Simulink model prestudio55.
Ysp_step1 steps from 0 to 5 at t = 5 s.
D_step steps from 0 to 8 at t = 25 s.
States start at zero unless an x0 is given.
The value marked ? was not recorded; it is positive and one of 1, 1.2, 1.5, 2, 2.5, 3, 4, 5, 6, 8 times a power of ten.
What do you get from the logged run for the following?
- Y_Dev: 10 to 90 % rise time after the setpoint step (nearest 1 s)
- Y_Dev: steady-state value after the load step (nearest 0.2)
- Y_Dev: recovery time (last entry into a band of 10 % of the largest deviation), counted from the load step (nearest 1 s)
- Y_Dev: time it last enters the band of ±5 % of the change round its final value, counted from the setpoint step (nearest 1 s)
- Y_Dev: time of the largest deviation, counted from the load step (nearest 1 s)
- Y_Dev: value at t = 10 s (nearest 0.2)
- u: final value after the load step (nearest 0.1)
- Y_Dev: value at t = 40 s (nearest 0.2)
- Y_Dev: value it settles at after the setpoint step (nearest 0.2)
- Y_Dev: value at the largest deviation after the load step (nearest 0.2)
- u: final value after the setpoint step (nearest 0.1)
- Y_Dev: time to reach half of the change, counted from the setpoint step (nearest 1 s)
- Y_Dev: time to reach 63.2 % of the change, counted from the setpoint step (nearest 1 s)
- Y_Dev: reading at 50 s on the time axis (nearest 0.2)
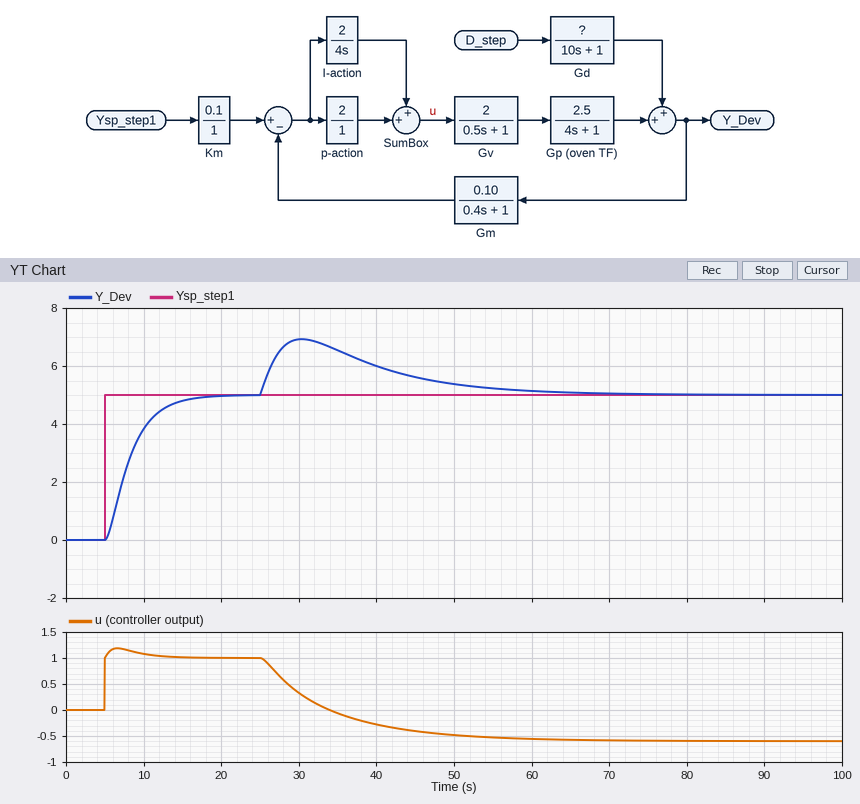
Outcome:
7 s
5.0
32 s
9 s
5 s
3.8
-0.6
6.0
5.0
7.0
1.0
3 s
4 s
5.4
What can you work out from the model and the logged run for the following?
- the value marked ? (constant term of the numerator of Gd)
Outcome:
1
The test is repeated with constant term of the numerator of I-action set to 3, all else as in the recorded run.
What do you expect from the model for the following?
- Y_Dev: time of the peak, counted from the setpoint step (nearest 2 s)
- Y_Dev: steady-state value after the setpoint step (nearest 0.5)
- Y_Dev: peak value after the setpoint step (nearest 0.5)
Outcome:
10 s
5.0
5.5
